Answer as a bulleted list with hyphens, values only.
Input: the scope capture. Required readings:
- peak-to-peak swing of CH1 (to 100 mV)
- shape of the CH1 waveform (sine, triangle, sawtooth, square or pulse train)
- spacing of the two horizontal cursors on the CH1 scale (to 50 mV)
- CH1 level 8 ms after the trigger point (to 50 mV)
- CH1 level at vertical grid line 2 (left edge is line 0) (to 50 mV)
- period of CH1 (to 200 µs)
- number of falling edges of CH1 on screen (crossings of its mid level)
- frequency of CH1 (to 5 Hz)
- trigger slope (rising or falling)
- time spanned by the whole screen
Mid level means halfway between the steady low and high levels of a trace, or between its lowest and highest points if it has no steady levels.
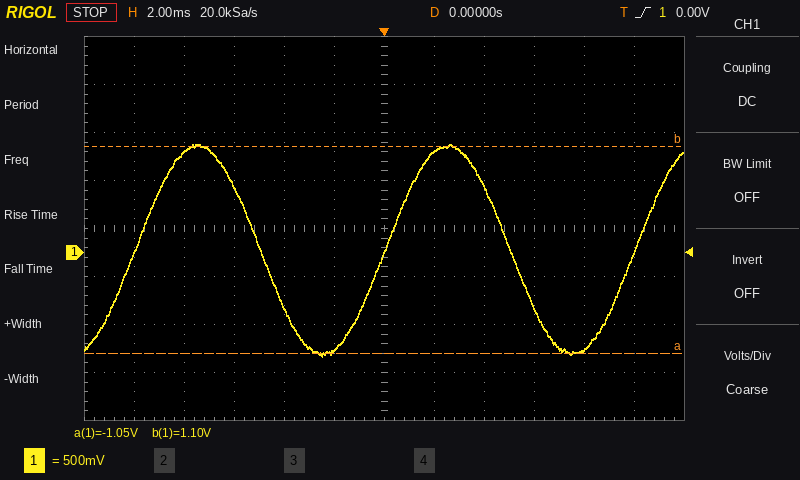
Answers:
- 2.20 V
- sine
- 2.15 V
- -1.00 V
- 1.05 V
- 10.0 ms
- 2
- 100 Hz
- rising
- 24 ms
